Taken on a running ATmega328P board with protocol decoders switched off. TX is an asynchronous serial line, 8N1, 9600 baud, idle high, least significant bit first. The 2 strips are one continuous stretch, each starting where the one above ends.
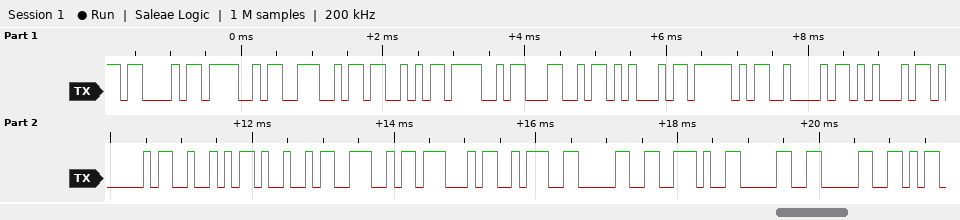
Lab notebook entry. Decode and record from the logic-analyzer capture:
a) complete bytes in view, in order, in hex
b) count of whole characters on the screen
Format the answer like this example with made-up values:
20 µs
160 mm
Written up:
43 4F 4E 53 4F 4C 45 5F 42 45 41 52 49 4E 47 3A 30 2E 30 30
20
